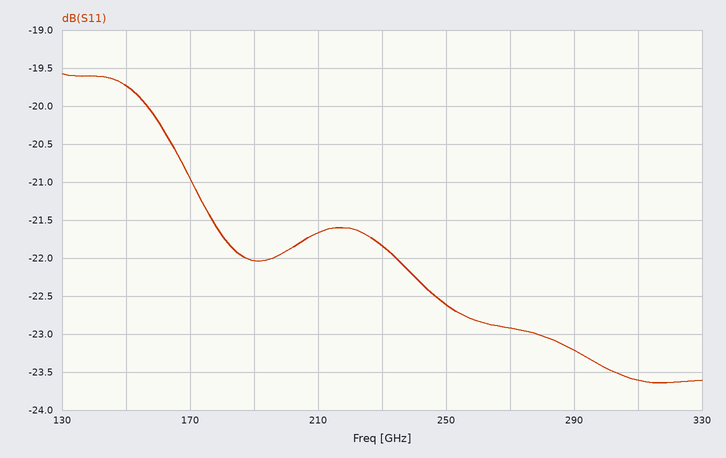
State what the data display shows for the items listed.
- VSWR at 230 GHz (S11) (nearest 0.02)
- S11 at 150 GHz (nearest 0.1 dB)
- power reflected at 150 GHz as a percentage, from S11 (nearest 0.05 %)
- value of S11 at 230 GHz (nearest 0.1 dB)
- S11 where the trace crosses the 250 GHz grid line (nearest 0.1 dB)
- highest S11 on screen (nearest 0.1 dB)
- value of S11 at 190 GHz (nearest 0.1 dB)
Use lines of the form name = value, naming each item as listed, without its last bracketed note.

VSWR at 230 GHz (S11) = 1.18
S11 at 150 GHz = -19.7 dB
power reflected at 150 GHz as a percentage, from S11 = 1.05 %
value of S11 at 230 GHz = -21.8 dB
S11 where the trace crosses the 250 GHz grid line = -22.6 dB
highest S11 on screen = -19.6 dB
value of S11 at 190 GHz = -22.0 dB
